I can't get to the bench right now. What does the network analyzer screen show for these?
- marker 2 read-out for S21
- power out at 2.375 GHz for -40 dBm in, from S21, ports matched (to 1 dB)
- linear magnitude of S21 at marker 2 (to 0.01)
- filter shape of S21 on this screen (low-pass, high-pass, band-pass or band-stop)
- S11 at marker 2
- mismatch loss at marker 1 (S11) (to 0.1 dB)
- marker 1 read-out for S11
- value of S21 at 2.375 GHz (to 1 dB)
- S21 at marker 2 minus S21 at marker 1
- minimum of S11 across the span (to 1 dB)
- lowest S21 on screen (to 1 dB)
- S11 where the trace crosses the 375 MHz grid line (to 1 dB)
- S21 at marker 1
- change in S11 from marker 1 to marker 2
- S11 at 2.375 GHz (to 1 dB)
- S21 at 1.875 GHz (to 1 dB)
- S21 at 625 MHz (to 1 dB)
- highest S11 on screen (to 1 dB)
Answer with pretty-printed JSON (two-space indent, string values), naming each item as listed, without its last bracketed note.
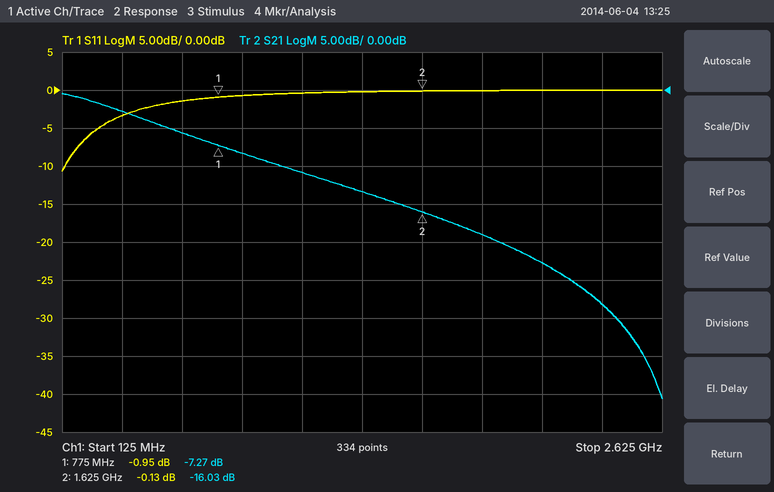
{
  "marker 2 read-out for S21": "-16.03 dB",
  "power out at 2.375 GHz for -40 dBm in, from S21, ports matched": "-68 dBm",
  "linear magnitude of S21 at marker 2": "0.16",
  "filter shape of S21 on this screen": "low-pass",
  "S11 at marker 2": "-0.13 dB",
  "mismatch loss at marker 1 (S11)": "7.1 dB",
  "marker 1 read-out for S11": "-0.95 dB",
  "value of S21 at 2.375 GHz": "-28 dB",
  "S21 at marker 2 minus S21 at marker 1": "-8.76 dB",
  "minimum of S11 across the span": "-11 dB",
  "lowest S21 on screen": "-41 dB",
  "S11 where the trace crosses the 375 MHz grid line": "-3 dB",
  "S21 at marker 1": "-7.27 dB",
  "change in S11 from marker 1 to marker 2": "0.82 dB",
  "S11 at 2.375 GHz": "0 dB",
  "S21 at 1.875 GHz": "-19 dB",
  "S21 at 625 MHz": "-6 dB",
  "highest S11 on screen": "0 dB"
}
